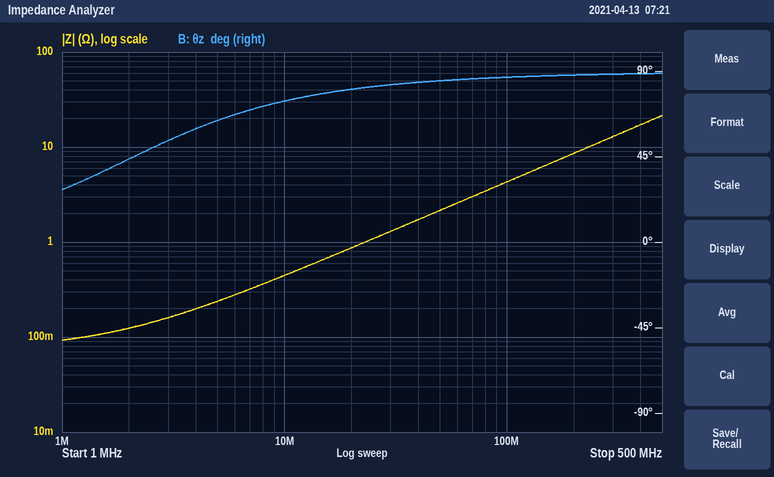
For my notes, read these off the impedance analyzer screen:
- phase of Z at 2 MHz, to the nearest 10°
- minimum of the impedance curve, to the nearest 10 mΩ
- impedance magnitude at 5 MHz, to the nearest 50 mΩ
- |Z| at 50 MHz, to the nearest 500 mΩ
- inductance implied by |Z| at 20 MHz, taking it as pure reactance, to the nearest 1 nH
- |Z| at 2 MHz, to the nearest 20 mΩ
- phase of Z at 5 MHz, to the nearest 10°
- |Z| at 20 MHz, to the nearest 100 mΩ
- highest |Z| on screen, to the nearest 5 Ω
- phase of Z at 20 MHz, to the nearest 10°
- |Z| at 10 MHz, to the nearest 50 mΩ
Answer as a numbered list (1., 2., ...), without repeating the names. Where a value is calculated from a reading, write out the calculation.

1. 40°
2. 90 mΩ
3. 250 mΩ
4. 2.0 Ω
5. L = 900 mΩ/(2π × 20 MHz) ≈ 7 nH
6. 120 mΩ
7. 60°
8. 900 mΩ
9. 20 Ω
10. 80°
11. 450 mΩ
